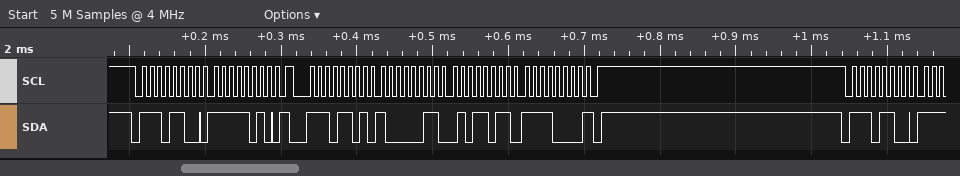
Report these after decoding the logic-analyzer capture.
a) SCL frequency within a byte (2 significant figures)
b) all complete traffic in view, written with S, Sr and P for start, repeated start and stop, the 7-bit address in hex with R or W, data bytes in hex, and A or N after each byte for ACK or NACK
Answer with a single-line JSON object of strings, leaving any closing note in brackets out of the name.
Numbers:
{"SCL frequency within a byte": "100 kHz", "all complete traffic in view, written with S, Sr and P for start, repeated start and stop, the 7-bit address in hex with R or W, data bytes in hex, and A or N after each byte for ACK or NACK": "S 76W A FA A Sr 76R A 83 A 5B A F0 N P S 76W A"}
